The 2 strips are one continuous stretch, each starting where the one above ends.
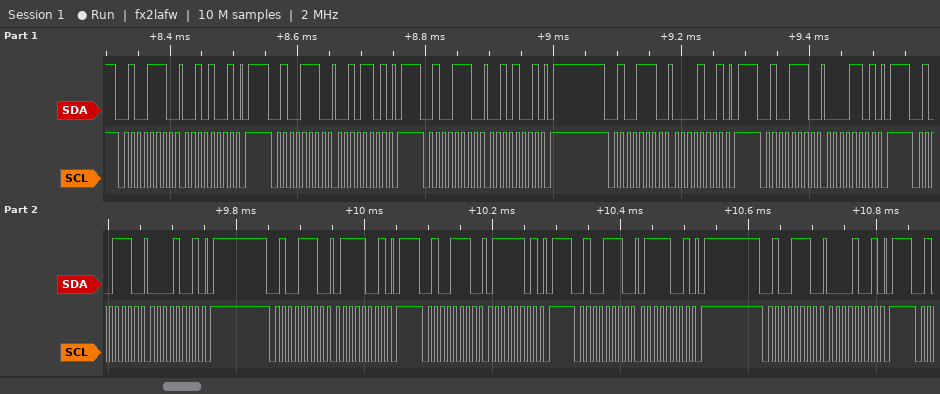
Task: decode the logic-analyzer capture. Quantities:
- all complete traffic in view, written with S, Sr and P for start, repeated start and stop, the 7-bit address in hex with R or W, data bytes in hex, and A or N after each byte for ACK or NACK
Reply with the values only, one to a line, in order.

S 27W A 29 A P S 27W A 2D A P S 27W A 29 A P S 27W A 09 A P S 27W A 0D A P S 27W A 09 A P S 27W A 79 A P S 27W A 7D A P S 27W A 79 A P S 27W A 09 A P
